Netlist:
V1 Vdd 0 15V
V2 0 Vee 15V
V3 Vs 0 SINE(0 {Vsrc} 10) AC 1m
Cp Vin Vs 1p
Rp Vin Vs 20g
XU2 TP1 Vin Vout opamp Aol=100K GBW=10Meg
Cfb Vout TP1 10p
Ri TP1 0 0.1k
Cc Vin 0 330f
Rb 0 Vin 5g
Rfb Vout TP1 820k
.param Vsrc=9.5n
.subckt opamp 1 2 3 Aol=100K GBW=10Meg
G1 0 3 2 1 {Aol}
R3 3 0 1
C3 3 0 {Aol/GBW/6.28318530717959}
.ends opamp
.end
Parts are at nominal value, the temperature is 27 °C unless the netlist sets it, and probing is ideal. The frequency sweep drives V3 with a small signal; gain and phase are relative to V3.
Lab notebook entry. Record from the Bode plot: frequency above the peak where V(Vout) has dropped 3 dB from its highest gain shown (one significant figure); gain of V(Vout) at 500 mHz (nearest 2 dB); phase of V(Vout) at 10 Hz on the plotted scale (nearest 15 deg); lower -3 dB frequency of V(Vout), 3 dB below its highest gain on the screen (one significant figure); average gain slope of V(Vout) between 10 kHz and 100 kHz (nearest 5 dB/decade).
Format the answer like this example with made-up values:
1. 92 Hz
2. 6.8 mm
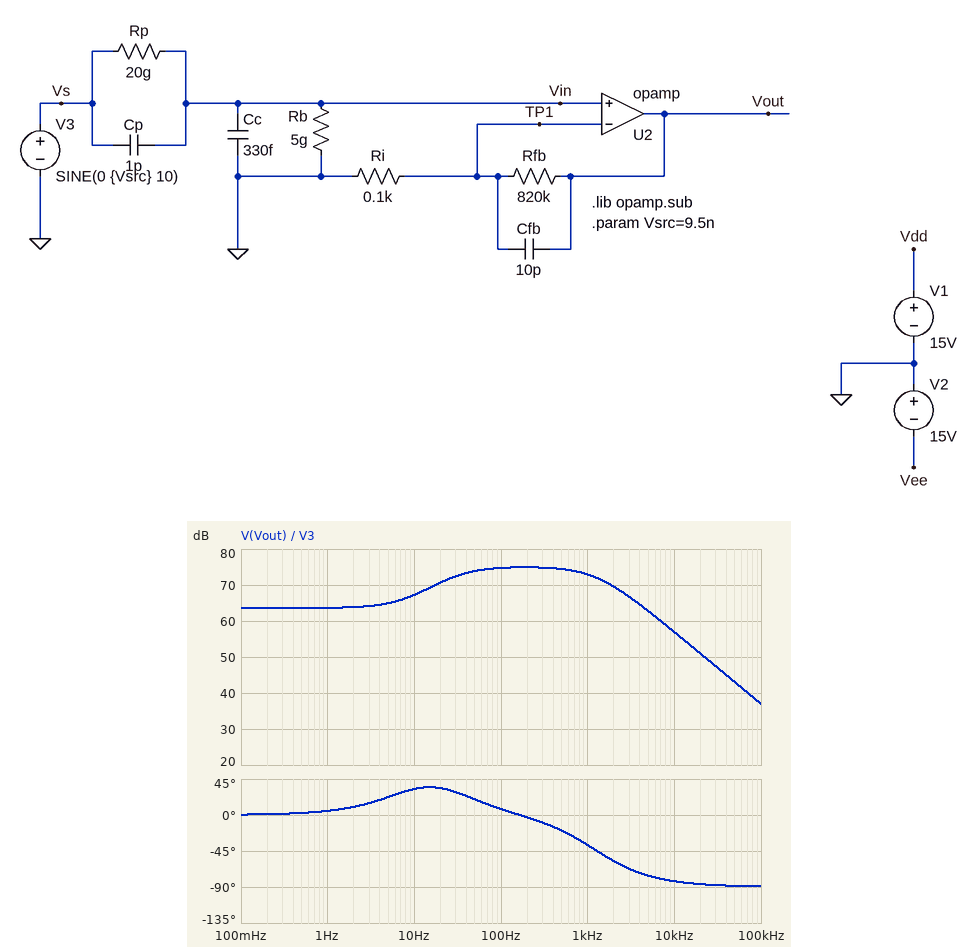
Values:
1. 1 kHz
2. 64 dB
3. 30 deg
4. 30 Hz
5. -20 dB/decade
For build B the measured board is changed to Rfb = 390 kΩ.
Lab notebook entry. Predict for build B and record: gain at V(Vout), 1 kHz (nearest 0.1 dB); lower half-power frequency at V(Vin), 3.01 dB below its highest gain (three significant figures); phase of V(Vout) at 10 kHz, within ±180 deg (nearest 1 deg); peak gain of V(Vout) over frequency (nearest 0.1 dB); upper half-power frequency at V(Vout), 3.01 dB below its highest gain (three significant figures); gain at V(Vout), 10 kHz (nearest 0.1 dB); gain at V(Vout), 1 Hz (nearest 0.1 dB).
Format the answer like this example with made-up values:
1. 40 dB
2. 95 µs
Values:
1. 68.4 dB
2. 27.7 Hz
3. -76 deg
4. 68.9 dB
5. 2.56 kHz
6. 56.7 dB
7. 57.6 dB
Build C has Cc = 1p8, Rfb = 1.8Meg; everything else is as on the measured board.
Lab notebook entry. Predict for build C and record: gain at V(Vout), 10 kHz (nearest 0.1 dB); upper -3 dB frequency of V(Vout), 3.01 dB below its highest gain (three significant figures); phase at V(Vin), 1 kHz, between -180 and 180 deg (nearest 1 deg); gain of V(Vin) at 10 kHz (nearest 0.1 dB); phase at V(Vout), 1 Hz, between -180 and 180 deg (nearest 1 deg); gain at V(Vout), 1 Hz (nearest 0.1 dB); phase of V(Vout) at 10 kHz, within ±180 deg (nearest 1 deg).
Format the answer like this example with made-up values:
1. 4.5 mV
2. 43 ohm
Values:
1. 50.5 dB
2. 640 Hz
3. 0 deg
4. -8.9 dB
5. 3 deg
6. 69.7 dB
7. -86 deg
